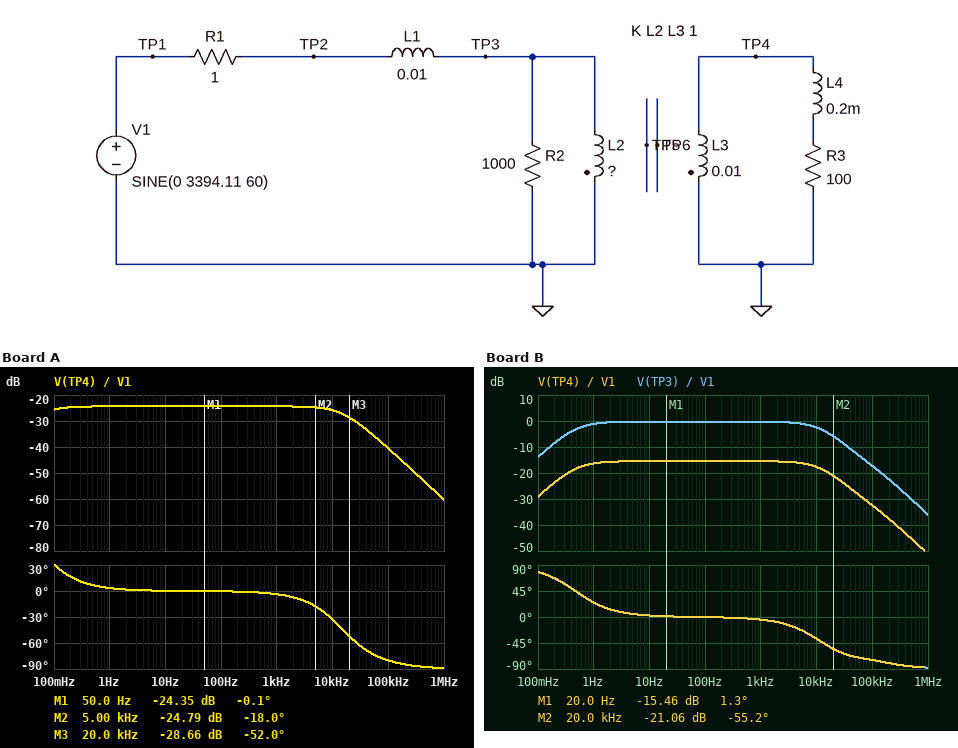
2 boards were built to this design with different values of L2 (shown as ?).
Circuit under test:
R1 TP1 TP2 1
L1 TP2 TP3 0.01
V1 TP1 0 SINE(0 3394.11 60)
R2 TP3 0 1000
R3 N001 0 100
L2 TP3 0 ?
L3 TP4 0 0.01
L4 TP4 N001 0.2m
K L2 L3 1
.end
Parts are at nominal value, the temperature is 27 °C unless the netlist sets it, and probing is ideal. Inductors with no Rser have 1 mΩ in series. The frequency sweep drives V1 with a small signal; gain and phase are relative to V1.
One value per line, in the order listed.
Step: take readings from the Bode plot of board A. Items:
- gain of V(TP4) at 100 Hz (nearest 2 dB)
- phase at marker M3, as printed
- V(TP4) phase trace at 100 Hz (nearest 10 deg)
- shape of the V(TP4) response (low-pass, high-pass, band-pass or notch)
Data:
-24 dB
-52.0 deg
0 deg
low-pass
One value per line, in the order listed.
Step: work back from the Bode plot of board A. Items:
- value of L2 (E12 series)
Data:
2.7 H
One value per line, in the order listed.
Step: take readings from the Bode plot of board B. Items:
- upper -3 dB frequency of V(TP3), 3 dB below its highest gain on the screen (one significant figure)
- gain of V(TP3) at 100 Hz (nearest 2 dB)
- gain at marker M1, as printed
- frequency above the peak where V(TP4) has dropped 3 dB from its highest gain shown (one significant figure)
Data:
10 kHz
0 dB
-15.46 dB
10 kHz
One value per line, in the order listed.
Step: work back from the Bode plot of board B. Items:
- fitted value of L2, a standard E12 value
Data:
330 mH
